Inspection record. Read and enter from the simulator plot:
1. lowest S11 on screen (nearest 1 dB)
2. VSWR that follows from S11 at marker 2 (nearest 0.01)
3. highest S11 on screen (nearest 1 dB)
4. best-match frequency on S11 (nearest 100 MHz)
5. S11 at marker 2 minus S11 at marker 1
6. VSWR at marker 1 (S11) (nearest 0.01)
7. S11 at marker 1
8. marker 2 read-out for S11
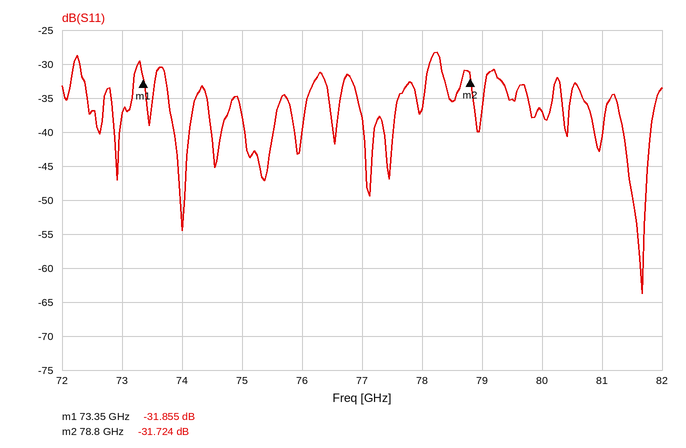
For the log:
-64 dB
1.05
-28 dB
81.7 GHz
0.131 dB
1.05
-31.855 dB
-31.724 dB
